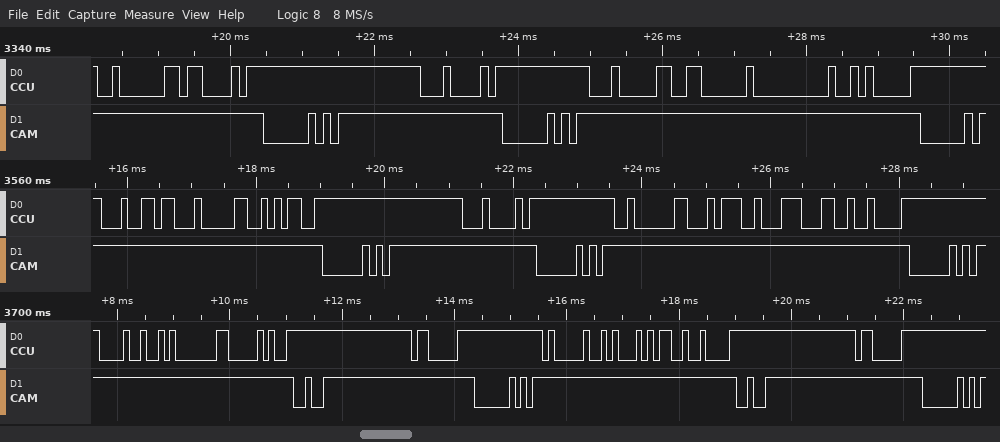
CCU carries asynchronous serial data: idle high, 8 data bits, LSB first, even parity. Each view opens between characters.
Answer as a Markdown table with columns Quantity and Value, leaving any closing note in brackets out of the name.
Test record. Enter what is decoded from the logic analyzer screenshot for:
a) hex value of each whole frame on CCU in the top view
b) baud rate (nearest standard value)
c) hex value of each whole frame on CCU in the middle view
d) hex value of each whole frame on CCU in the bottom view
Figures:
| Quantity | Value |
|---|---|
| hex value of each whole frame on CCU in the top view | 02, 43, 84, 04, 06, 00, 0A |
| baud rate | 9600 baud |
| hex value of each whole frame on CCU in the middle view | 64, 04, 6A, 84, 02, 74, 1C, 12 |
| hex value of each whole frame on CCU in the bottom view | 48, 01, 50, 83, 41, 51, 12, 83 |
